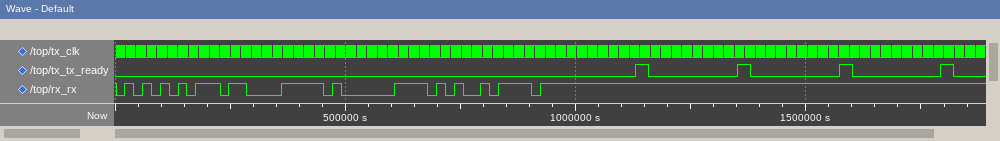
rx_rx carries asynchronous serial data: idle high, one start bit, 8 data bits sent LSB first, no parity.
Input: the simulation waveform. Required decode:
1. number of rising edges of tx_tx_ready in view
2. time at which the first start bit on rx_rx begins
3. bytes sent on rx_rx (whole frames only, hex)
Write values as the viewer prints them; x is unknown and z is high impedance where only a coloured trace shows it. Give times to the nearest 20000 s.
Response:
4
0 s
55, C3, 81, A5, FF
